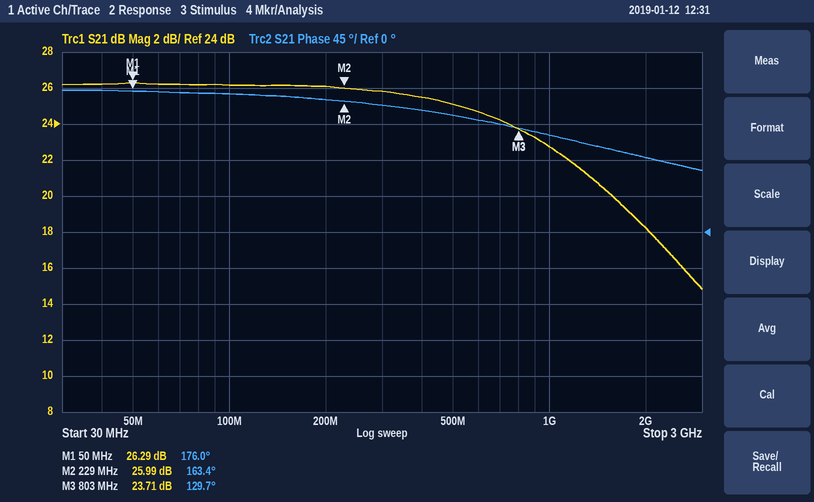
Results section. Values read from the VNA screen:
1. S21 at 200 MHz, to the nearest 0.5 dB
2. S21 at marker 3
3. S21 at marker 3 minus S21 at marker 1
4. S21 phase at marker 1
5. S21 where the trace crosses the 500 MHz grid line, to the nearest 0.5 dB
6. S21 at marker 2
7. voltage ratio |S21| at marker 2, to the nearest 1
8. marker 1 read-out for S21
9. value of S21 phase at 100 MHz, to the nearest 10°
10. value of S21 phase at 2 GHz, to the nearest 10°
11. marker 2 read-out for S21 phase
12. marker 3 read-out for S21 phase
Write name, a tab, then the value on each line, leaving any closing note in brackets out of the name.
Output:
S21 at 200 MHz, to the nearest 0.5 dB	26.0 dB
S21 at marker 3	23.71 dB
S21 at marker 3 minus S21 at marker 1	-2.58 dB
S21 phase at marker 1	176.0°
S21 where the trace crosses the 500 MHz grid line, to the nearest 0.5 dB	25.0 dB
S21 at marker 2	25.99 dB
voltage ratio |S21| at marker 2, to the nearest 1	20
marker 1 read-out for S21	26.29 dB
value of S21 phase at 100 MHz, to the nearest 10°	170°
value of S21 phase at 2 GHz, to the nearest 10°	90°
marker 2 read-out for S21 phase	163.4°
marker 3 read-out for S21 phase	129.7°
